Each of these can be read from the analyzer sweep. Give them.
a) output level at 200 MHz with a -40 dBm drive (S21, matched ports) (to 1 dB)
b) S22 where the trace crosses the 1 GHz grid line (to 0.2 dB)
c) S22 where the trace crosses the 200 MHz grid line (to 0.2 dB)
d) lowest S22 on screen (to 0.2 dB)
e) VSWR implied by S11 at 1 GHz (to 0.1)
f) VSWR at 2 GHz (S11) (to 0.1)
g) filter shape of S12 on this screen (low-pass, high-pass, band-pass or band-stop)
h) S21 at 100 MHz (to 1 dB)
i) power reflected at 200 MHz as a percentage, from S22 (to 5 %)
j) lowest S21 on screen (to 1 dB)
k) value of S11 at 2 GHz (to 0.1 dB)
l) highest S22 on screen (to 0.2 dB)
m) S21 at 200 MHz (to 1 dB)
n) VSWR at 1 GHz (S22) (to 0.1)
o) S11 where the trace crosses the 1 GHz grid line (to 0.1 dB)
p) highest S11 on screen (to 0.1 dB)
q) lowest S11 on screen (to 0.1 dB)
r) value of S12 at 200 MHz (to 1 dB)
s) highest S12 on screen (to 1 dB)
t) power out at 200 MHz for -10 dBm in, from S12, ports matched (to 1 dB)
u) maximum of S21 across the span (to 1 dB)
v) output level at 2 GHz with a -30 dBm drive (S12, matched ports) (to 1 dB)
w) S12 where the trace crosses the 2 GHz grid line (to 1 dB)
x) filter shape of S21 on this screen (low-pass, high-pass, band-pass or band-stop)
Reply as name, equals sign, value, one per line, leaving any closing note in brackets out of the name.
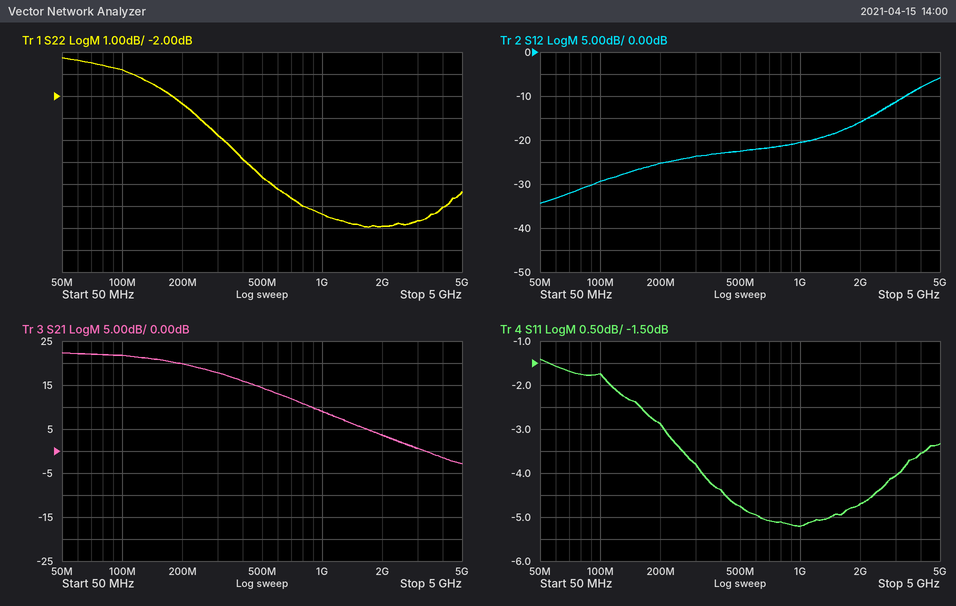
output level at 200 MHz with a -40 dBm drive (S21, matched ports) = -20 dBm
S22 where the trace crosses the 1 GHz grid line = -7.4 dB
S22 where the trace crosses the 200 MHz grid line = -2.4 dB
lowest S22 on screen = -8.0 dB
VSWR implied by S11 at 1 GHz = 3.4
VSWR at 2 GHz (S11) = 3.8
filter shape of S12 on this screen = high-pass
S21 at 100 MHz = 22 dB
power reflected at 200 MHz as a percentage, from S22 = 60 %
lowest S21 on screen = -3 dB
value of S11 at 2 GHz = -4.7 dB
highest S22 on screen = -0.2 dB
S21 at 200 MHz = 20 dB
VSWR at 1 GHz (S22) = 2.5
S11 where the trace crosses the 1 GHz grid line = -5.2 dB
highest S11 on screen = -1.4 dB
lowest S11 on screen = -5.2 dB
value of S12 at 200 MHz = -25 dB
highest S12 on screen = -6 dB
power out at 200 MHz for -10 dBm in, from S12, ports matched = -35 dBm
maximum of S21 across the span = 22 dB
output level at 2 GHz with a -30 dBm drive (S12, matched ports) = -46 dBm
S12 where the trace crosses the 2 GHz grid line = -16 dB
filter shape of S21 on this screen = low-pass
